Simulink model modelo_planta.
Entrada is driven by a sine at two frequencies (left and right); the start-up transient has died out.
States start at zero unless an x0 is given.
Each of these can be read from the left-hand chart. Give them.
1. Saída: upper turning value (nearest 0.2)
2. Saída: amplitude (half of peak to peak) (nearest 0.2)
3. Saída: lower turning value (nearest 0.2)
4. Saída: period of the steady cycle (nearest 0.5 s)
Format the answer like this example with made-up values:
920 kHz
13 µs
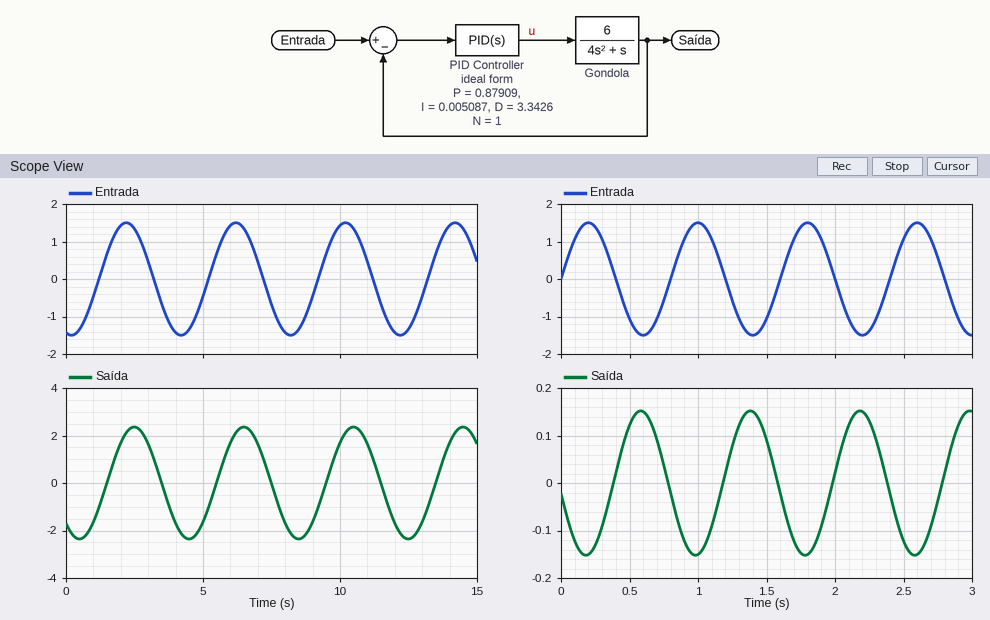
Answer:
2.4
2.4
-2.4
4.0 s
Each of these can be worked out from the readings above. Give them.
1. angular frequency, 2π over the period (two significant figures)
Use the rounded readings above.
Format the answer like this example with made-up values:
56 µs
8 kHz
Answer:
1.6 rad/s
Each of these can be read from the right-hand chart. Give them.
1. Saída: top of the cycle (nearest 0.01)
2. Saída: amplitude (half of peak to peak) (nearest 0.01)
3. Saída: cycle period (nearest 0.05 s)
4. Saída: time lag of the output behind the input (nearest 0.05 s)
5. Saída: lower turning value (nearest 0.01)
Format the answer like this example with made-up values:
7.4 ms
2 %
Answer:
0.15
0.15
0.80 s
0.40 s
-0.15
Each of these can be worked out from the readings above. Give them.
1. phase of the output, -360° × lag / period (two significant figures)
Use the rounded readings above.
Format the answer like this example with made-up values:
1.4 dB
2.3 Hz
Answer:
-180°
